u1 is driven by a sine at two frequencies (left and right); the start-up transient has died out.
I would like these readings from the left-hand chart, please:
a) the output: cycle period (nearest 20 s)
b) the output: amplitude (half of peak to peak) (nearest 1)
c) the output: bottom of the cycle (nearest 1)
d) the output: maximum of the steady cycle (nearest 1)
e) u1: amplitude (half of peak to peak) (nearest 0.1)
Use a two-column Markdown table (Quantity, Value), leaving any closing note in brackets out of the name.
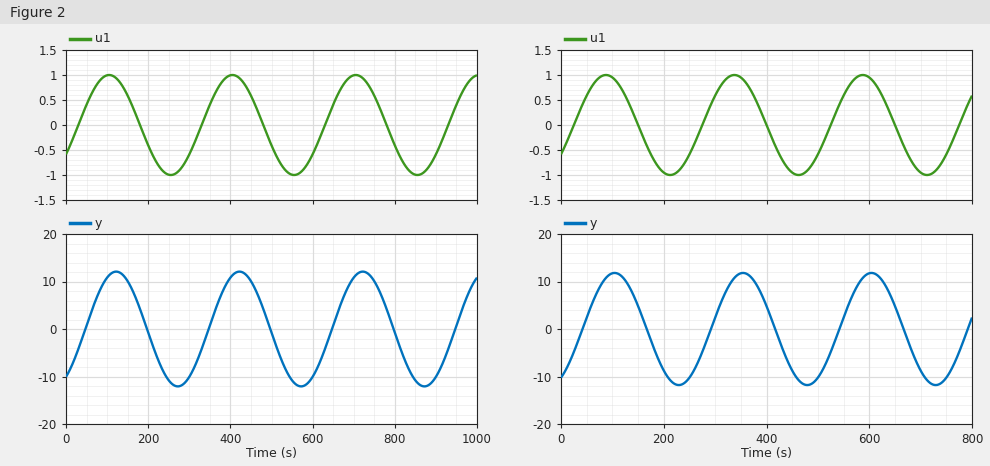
| Quantity | Value |
|---|---|
| the output: cycle period | 300 s |
| the output: amplitude (half of peak to peak) | 12 |
| the output: bottom of the cycle | -12 |
| the output: maximum of the steady cycle | 12 |
| u1: amplitude (half of peak to peak) | 1.0 |
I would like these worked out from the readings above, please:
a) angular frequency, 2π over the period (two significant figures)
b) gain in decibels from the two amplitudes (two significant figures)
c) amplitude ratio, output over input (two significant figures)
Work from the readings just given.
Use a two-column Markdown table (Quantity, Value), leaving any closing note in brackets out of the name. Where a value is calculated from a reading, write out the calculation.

| Quantity | Value |
|---|---|
| angular frequency, 2π over the period | 2π / 300 = 0.021 rad/s |
| gain in decibels from the two amplitudes | 20 log10(12 / 1) = 22 dB |
| amplitude ratio, output over input | 12 / 1 = 12 |
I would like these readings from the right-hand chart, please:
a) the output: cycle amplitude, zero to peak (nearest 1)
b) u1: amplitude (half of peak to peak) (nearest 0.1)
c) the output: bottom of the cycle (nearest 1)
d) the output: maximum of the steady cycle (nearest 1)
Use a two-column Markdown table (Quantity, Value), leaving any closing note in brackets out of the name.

| Quantity | Value |
|---|---|
| the output: cycle amplitude, zero to peak | 12 |
| u1: amplitude (half of peak to peak) | 1.0 |
| the output: bottom of the cycle | -12 |
| the output: maximum of the steady cycle | 12 |
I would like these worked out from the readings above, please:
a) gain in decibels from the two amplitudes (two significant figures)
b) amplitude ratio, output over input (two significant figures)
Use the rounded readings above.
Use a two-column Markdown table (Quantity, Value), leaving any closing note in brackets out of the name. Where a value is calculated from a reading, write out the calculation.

| Quantity | Value |
|---|---|
| gain in decibels from the two amplitudes | 20 log10(12 / 1) = 22 dB |
| amplitude ratio, output over input | 12 / 1 = 12 |
